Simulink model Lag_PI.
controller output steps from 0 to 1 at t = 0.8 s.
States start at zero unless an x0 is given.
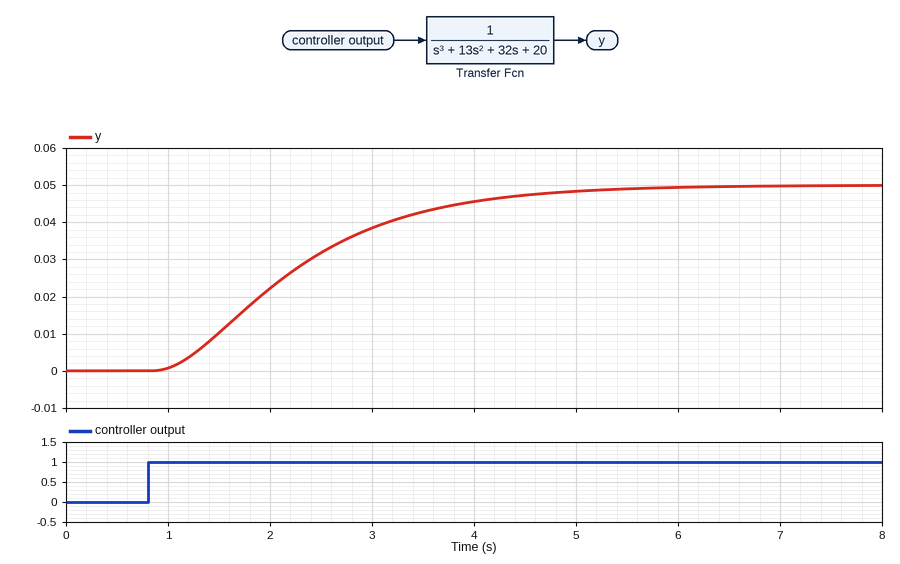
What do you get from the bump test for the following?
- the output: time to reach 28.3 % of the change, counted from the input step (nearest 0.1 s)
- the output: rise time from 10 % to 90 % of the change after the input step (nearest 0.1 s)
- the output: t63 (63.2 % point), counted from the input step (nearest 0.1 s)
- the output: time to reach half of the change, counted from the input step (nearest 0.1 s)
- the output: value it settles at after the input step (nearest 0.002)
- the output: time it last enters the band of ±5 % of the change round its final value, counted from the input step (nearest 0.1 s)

0.9 s
2.6 s
1.7 s
1.3 s
0.050
3.8 s
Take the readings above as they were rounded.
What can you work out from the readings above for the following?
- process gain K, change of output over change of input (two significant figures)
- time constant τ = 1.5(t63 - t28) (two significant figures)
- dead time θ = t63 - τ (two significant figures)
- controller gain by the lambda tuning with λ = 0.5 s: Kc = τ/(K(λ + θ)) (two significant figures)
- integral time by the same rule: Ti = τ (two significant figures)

0.050
1.2 s
0.50 s
24
1.2 s
